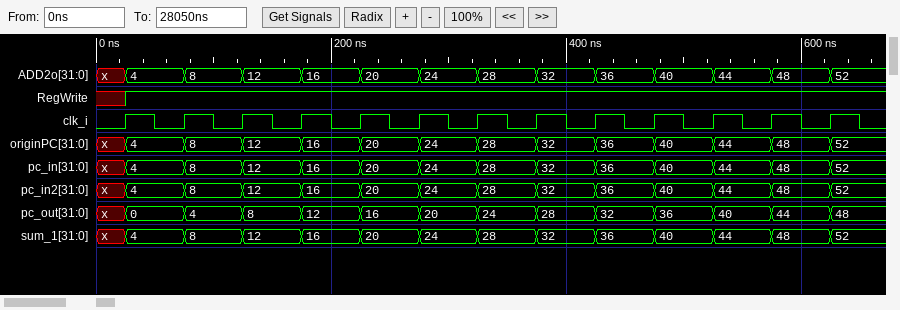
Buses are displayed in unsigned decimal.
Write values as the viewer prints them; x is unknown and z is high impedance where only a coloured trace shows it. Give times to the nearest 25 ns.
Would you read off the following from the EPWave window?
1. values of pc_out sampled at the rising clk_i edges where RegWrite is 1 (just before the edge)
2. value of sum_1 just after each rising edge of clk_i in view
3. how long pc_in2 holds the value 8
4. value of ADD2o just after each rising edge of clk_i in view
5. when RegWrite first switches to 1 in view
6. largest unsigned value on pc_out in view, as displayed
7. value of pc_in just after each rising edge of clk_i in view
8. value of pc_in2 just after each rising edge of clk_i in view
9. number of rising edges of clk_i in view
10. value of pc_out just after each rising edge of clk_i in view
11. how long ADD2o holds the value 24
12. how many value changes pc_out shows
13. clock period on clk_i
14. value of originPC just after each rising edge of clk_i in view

0, 4, 8, 12, 16, 20, 24, 28, 32, 36, 40, 44
4, 8, 12, 16, 20, 24, 28, 32, 36, 40, 44, 48, 52
50 ns
4, 8, 12, 16, 20, 24, 28, 32, 36, 40, 44, 48, 52
25 ns
48
4, 8, 12, 16, 20, 24, 28, 32, 36, 40, 44, 48, 52
4, 8, 12, 16, 20, 24, 28, 32, 36, 40, 44, 48, 52
13
0, 4, 8, 12, 16, 20, 24, 28, 32, 36, 40, 44, 48
50 ns
13
50 ns
4, 8, 12, 16, 20, 24, 28, 32, 36, 40, 44, 48, 52
